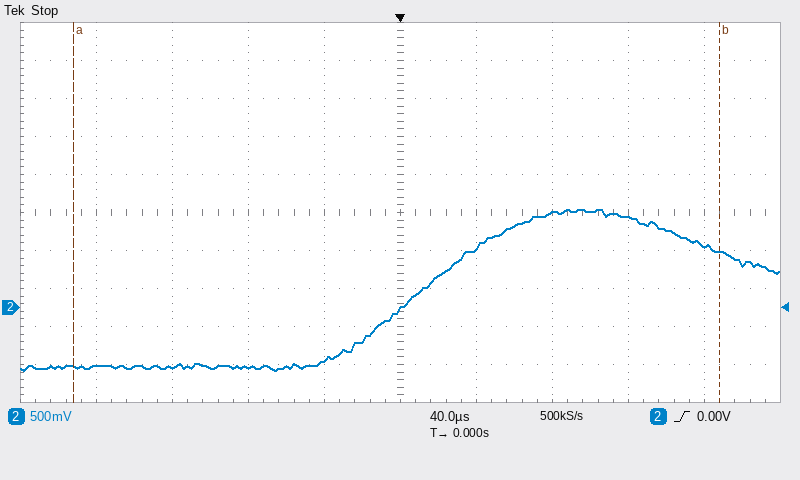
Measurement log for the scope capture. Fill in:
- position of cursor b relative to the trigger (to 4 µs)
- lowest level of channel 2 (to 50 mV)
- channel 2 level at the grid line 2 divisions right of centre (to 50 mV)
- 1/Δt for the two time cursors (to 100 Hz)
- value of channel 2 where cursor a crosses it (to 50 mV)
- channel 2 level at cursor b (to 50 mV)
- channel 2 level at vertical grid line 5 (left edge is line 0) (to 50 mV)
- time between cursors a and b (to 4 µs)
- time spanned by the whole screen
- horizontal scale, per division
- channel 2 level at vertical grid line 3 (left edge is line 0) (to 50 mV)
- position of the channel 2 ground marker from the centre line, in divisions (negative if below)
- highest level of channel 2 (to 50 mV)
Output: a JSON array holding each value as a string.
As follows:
["+168 µs", "-850 mV", "1.25 V", "2.9 kHz", "-800 mV", "750 mV", "-50 mV", "340 µs", "400 µs", "40 µs", "-800 mV", "-2.5 div", "1.30 V"]
